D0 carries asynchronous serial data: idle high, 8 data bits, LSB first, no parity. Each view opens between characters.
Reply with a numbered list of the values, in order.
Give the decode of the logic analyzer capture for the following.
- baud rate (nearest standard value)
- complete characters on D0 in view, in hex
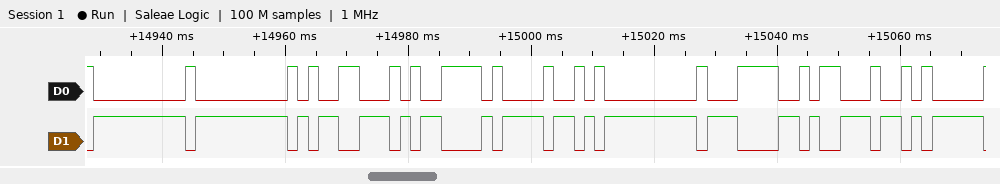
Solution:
1. 600 baud
2. 00, 00, 19, 79, 48, 00, 3C, 23
